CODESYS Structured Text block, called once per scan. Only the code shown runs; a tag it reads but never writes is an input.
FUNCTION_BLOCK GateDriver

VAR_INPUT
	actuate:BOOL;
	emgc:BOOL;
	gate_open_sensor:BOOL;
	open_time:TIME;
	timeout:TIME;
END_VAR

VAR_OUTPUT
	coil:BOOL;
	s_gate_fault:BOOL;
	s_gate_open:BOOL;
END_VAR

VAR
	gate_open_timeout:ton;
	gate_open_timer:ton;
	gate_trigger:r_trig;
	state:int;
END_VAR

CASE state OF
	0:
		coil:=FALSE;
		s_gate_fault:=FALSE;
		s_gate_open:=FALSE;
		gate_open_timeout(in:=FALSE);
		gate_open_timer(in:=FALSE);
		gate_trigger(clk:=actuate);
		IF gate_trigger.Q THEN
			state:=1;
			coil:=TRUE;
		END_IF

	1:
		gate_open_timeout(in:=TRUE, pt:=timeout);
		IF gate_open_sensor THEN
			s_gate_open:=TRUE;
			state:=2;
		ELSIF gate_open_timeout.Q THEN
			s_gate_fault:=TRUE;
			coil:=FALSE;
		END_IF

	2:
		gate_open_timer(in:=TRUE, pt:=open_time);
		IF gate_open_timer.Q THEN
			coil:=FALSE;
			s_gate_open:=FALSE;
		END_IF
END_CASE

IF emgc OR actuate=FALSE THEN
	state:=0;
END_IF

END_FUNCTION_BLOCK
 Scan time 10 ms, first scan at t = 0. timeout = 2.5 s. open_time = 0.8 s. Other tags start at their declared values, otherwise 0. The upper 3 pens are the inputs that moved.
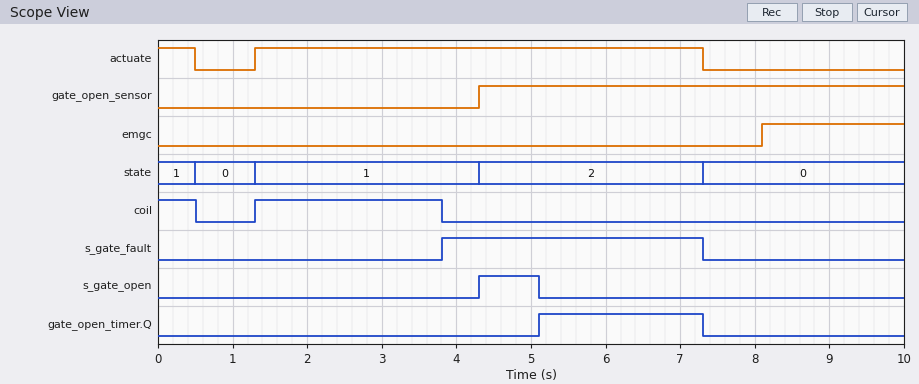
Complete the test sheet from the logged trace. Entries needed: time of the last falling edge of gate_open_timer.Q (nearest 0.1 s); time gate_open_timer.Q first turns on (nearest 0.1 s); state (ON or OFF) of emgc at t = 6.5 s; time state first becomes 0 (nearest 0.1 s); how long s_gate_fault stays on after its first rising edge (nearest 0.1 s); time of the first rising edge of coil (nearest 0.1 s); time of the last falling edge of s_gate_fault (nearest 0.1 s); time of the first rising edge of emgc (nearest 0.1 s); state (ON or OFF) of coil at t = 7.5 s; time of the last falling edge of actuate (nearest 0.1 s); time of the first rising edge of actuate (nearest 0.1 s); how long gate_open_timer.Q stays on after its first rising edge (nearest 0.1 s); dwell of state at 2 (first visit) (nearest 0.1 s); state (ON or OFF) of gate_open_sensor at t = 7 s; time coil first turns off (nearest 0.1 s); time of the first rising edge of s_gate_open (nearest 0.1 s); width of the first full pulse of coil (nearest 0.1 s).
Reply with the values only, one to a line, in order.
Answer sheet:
7.3 s
5.1 s
OFF
0.5 s
3.5 s
1.3 s
7.3 s
8.1 s
OFF
7.3 s
1.3 s
2.2 s
3.0 s
ON
0.5 s
4.3 s
2.5 s
